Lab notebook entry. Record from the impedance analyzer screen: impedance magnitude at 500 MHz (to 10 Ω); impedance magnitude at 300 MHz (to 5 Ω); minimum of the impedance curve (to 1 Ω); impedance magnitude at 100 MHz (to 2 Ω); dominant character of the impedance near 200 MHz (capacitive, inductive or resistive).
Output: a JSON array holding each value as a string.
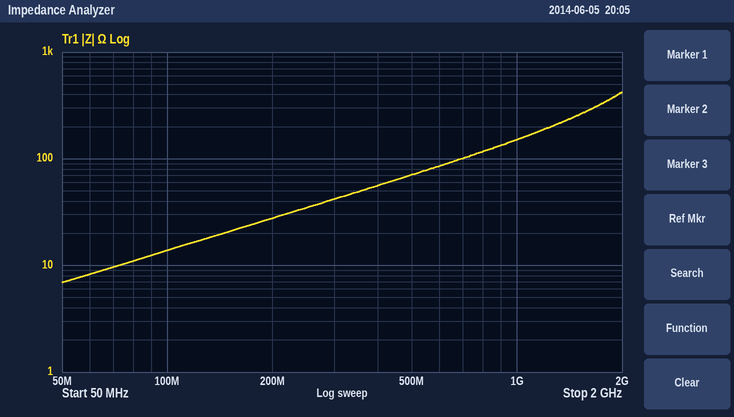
["70 Ω", "40 Ω", "7 Ω", "14 Ω", "inductive"]
